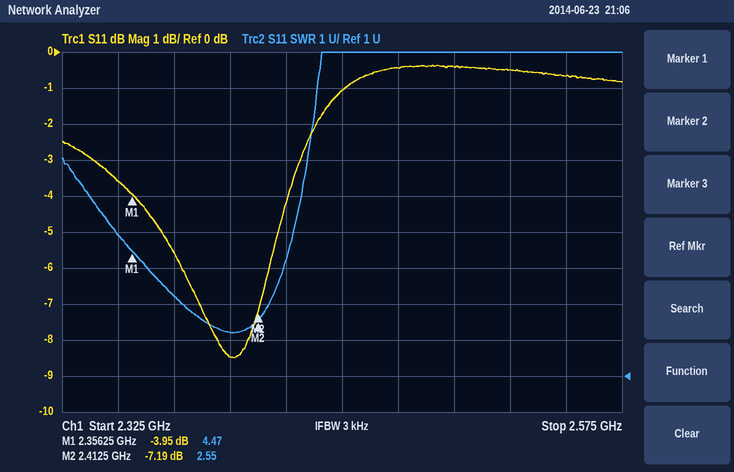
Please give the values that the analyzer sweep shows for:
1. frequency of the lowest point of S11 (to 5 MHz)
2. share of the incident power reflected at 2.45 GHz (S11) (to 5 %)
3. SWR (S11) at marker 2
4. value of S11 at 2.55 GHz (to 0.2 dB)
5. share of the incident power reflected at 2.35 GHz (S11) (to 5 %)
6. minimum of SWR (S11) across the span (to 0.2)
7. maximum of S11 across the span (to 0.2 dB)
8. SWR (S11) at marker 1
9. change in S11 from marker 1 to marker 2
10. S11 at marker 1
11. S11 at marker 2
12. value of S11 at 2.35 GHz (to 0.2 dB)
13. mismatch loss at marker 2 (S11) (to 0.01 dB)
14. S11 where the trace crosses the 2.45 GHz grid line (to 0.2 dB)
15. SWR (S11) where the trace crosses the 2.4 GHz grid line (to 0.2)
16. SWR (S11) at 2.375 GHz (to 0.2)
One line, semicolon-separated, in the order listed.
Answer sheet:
2.400 GHz; 80 %; 2.55; -0.6 dB; 45 %; 2.2; -0.4 dB; 4.47; -3.24 dB; -3.95 dB; -7.19 dB; -3.6 dB; 0.92 dB; -1.0 dB; 2.2; 3.2
